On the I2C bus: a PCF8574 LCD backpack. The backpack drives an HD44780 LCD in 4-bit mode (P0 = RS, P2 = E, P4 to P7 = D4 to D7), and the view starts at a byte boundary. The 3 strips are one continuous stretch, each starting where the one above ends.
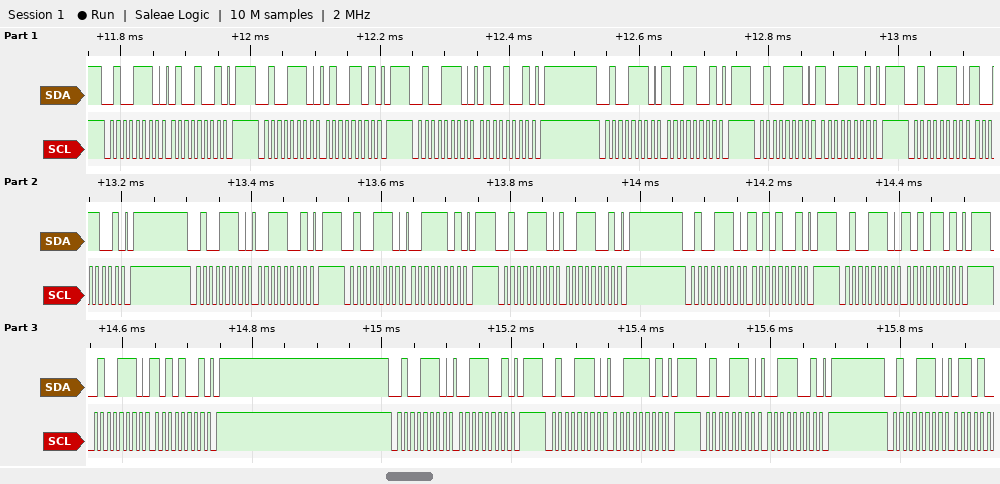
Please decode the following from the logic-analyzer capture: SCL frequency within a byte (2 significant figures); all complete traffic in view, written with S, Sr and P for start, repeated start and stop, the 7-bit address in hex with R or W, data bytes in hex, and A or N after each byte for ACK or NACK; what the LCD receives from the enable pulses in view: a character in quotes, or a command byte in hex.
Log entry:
100 kHz
S 27W A 49 A P S 27W A 4D A P S 27W A 49 A P S 27W A 99 A P S 27W A 9D A P S 27W A 99 A P S 27W A 39 A P S 27W A 3D A P S 27W A 39 A P S 27W A A9 A P S 27W A AD A P S 27W A A9 A P S 27W A 39 A P S 27W A 3D A P S 27W A 39 A P S 27W A
'I' ':'
